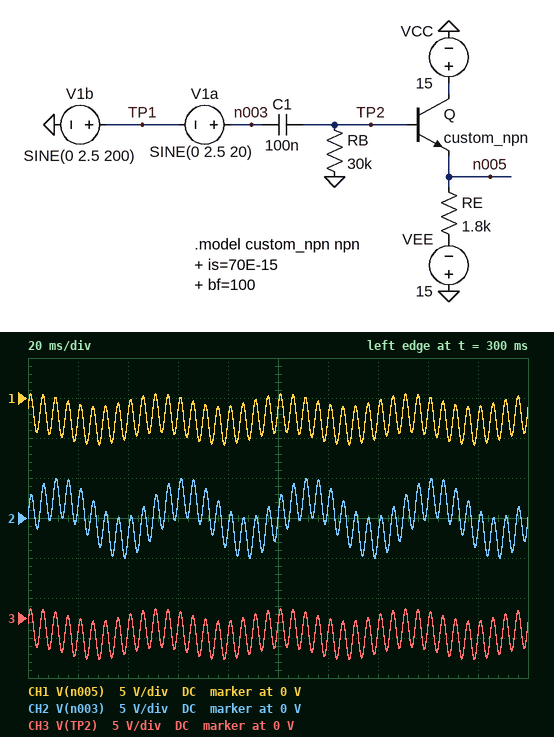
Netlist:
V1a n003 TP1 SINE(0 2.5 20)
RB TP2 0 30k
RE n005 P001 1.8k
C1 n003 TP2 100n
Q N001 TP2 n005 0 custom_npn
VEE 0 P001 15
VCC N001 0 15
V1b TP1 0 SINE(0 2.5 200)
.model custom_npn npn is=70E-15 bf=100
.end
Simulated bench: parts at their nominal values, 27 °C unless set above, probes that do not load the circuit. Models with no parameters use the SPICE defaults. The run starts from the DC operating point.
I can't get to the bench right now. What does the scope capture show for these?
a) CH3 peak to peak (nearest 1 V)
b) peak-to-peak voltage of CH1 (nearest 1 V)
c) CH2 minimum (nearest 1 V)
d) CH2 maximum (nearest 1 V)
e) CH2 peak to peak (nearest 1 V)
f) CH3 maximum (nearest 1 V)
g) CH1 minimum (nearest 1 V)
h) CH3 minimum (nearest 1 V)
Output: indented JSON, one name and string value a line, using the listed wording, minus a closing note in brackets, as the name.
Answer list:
{
  "CH3 peak to peak": "6 V",
  "peak-to-peak voltage of CH1": "6 V",
  "CH2 minimum": "-5 V",
  "CH2 maximum": "5 V",
  "CH2 peak to peak": "10 V",
  "CH3 maximum": "1 V",
  "CH1 minimum": "-6 V",
  "CH3 minimum": "-5 V"
}
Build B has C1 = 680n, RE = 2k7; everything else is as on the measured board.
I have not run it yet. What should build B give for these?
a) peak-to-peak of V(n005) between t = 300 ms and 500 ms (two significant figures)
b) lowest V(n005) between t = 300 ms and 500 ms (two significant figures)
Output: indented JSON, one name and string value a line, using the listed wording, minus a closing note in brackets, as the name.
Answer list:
{
  "peak-to-peak of V(n005) between t = 300 ms and 500 ms": "9.5 V",
  "lowest V(n005) between t = 300 ms and 500 ms": "-6.8 V"
}
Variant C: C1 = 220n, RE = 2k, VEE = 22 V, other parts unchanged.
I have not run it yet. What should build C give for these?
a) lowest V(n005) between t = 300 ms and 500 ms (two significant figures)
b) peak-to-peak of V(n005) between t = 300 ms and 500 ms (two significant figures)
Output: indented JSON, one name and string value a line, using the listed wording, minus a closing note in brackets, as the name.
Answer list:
{
  "lowest V(n005) between t = 300 ms and 500 ms": "-7.3 V",
  "peak-to-peak of V(n005) between t = 300 ms and 500 ms": "7.8 V"
}
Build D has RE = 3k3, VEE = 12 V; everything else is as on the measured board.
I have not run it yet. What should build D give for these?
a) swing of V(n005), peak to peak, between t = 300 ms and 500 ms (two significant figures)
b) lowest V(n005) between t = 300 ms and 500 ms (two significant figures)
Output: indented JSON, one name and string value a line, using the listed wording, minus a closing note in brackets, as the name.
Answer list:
{
  "swing of V(n005), peak to peak, between t = 300 ms and 500 ms": "6.4 V",
  "lowest V(n005) between t = 300 ms and 500 ms": "-4.8 V"
}
